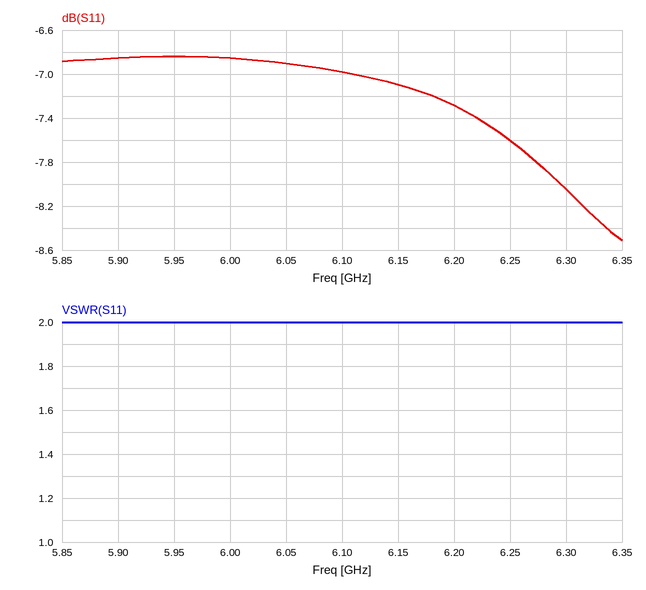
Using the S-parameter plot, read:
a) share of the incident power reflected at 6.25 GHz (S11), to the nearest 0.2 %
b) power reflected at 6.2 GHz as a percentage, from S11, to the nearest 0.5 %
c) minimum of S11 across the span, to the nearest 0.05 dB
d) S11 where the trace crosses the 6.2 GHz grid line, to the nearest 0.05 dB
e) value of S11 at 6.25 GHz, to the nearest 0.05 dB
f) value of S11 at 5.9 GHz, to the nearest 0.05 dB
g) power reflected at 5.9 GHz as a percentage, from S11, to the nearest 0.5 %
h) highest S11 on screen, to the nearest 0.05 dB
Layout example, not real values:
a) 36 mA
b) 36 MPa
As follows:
a) 17.4 %
b) 18.5 %
c) -8.50 dB
d) -7.30 dB
e) -7.60 dB
f) -6.85 dB
g) 20.5 %
h) -6.85 dB
